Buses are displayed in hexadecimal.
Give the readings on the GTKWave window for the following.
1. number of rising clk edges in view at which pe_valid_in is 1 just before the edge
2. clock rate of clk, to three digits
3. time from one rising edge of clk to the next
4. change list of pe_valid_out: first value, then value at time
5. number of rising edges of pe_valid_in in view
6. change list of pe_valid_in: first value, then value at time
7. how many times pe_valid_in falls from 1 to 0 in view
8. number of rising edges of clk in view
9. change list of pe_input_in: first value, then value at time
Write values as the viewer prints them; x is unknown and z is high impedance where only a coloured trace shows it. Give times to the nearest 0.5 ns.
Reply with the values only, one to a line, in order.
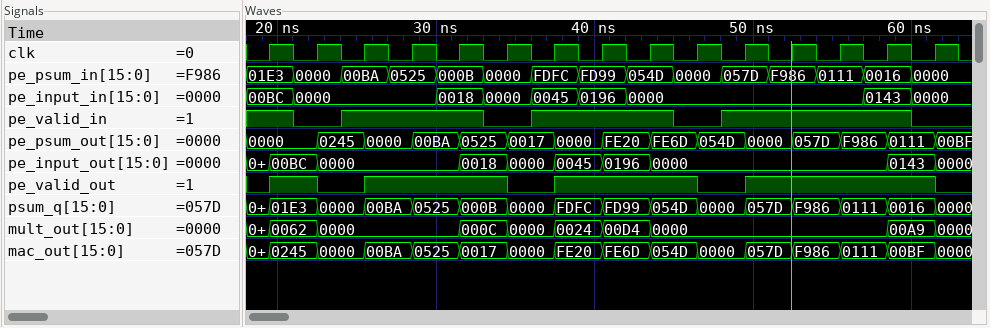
11
333 MHz
3 ns
0, 1 at 19.5 ns, 0 at 22.5 ns, 1 at 25.5 ns, 0 at 34.5 ns, 1 at 37.5 ns, 0 at 46.5 ns, 1 at 49.5 ns, 0 at 61.5 ns
3
1, 0 at 21 ns, 1 at 24 ns, 0 at 33 ns, 1 at 36 ns, 0 at 45 ns, 1 at 48 ns, 0 at 60 ns
4
15
00BC, 0000 at 21 ns, 0018 at 30 ns, 0000 at 33 ns, 0045 at 36 ns, 0196 at 39 ns, 0000 at 42 ns, 0143 at 57 ns, 0000 at 60 ns
